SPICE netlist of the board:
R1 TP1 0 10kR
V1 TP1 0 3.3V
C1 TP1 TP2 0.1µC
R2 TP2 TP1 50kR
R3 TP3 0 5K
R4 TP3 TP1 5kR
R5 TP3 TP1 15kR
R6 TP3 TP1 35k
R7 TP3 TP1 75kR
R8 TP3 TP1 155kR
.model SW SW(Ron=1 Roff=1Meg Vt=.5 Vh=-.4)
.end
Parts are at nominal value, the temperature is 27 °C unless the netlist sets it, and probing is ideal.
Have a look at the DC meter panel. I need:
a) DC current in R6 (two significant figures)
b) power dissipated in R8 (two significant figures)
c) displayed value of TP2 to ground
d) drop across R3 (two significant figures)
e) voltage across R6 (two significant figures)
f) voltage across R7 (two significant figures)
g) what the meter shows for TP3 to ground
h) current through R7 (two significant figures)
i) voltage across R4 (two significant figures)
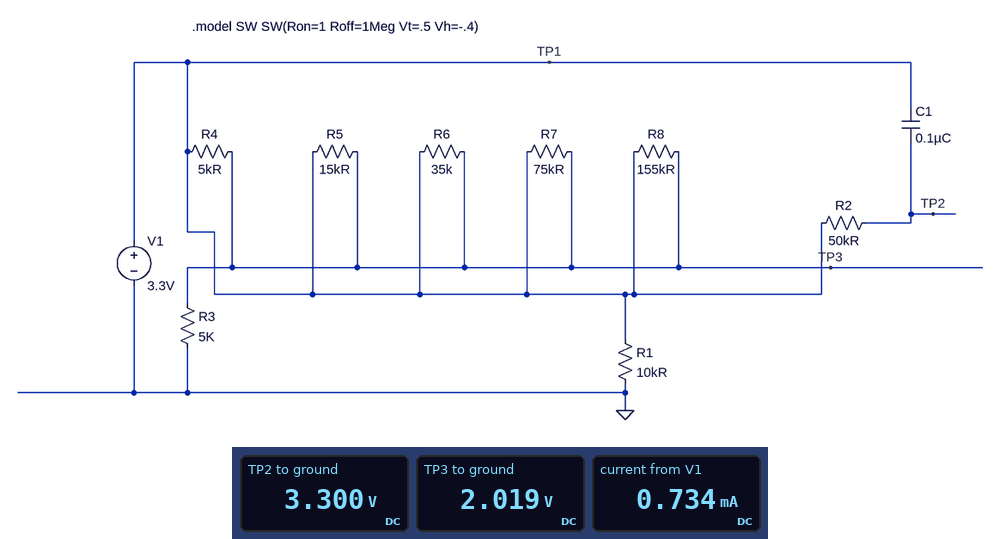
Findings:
37 µA
11 µW
3.300 V
2.0 V
1.3 V
1.3 V
2.019 V
17 µA
1.3 V
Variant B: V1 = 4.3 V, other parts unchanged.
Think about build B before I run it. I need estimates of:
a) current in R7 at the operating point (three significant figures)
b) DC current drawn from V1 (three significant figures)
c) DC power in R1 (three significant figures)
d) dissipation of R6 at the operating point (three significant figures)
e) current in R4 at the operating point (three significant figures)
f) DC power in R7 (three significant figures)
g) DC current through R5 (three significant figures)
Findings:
22.3 µA
956 µA
1.85 mW
79.7 µW
334 µA
37.2 µW
111 µA
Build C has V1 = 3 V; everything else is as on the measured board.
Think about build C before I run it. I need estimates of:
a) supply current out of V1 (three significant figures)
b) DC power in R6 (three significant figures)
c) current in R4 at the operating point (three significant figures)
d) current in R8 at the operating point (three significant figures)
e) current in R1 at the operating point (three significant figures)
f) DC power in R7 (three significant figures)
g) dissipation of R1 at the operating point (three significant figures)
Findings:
667 µA
38.8 µW
233 µA
7.52 µA
300 µA
18.1 µW
900 µW
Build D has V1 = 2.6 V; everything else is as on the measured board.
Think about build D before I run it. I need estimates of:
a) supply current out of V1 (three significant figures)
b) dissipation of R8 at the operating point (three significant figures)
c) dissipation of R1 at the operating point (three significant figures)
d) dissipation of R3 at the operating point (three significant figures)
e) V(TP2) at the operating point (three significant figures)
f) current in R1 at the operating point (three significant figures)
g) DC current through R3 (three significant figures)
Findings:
578 µA
6.58 µW
676 µW
506 µW
2.60 V
260 µA
318 µA
